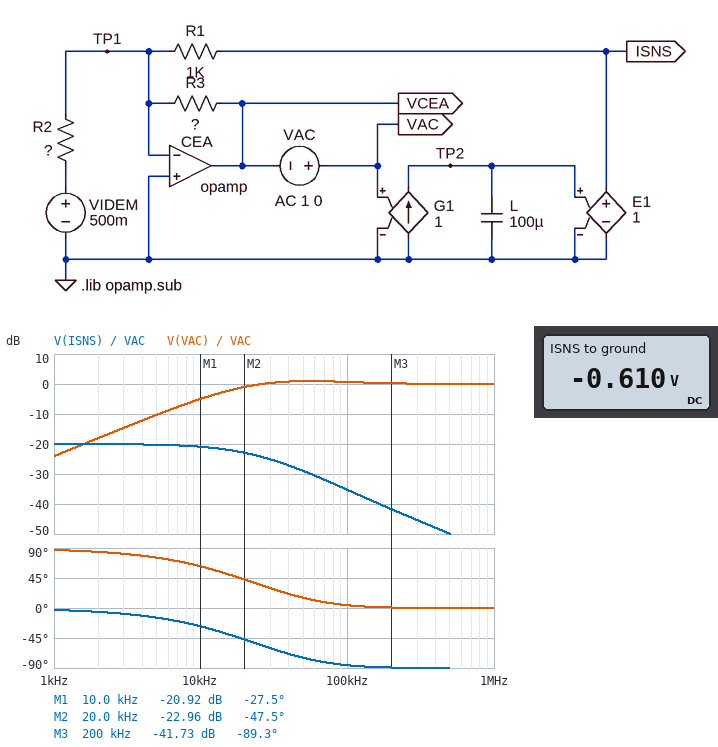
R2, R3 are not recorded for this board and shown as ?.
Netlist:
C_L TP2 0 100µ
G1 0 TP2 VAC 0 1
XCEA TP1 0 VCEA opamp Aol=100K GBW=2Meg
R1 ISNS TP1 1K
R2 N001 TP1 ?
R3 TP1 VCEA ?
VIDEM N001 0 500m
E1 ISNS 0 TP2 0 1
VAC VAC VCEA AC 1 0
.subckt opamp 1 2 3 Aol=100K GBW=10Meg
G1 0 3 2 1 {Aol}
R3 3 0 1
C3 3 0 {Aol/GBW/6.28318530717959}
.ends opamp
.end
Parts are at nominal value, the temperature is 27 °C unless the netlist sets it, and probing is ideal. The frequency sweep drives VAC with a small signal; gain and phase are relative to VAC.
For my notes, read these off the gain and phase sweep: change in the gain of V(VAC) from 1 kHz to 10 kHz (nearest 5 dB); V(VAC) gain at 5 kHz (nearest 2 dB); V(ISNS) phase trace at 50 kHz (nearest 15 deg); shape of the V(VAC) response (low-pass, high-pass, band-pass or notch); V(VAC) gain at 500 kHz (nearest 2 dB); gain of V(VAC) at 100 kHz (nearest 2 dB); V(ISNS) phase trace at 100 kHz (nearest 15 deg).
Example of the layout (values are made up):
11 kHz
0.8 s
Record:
20 dB
-10 dB
-75 deg
high-pass
0 dB
0 dB
-90 deg
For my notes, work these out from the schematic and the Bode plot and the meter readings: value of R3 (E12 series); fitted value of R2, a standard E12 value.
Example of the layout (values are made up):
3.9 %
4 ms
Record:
10 kΩ
820 Ω
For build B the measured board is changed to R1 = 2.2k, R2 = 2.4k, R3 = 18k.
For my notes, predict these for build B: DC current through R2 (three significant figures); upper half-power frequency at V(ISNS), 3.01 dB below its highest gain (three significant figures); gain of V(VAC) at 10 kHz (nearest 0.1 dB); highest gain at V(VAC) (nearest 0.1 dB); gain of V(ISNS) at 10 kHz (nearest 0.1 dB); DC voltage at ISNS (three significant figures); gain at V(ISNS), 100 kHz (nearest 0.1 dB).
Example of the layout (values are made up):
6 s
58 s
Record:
208 µA
14.8 kHz
-3.9 dB
0.6 dB
-19.9 dB
-458 mV
-35.4 dB
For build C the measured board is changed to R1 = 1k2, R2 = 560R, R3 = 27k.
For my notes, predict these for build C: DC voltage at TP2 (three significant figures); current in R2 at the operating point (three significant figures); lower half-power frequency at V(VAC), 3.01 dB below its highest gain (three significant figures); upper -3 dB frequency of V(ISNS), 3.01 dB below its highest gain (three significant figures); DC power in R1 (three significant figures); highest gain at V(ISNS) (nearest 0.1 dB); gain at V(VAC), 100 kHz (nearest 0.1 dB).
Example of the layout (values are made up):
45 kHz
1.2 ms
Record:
-1.07 V
893 µA
23.9 kHz
43.3 kHz
957 µW
-22.2 dB
0.8 dB
